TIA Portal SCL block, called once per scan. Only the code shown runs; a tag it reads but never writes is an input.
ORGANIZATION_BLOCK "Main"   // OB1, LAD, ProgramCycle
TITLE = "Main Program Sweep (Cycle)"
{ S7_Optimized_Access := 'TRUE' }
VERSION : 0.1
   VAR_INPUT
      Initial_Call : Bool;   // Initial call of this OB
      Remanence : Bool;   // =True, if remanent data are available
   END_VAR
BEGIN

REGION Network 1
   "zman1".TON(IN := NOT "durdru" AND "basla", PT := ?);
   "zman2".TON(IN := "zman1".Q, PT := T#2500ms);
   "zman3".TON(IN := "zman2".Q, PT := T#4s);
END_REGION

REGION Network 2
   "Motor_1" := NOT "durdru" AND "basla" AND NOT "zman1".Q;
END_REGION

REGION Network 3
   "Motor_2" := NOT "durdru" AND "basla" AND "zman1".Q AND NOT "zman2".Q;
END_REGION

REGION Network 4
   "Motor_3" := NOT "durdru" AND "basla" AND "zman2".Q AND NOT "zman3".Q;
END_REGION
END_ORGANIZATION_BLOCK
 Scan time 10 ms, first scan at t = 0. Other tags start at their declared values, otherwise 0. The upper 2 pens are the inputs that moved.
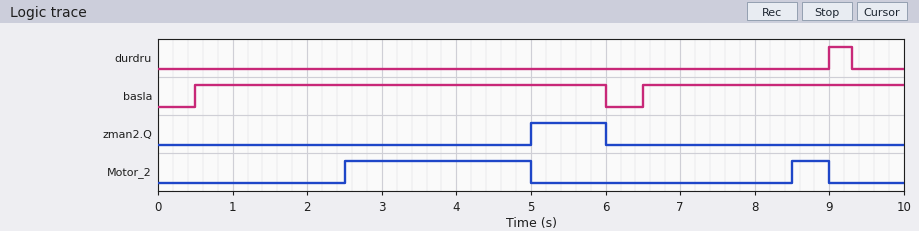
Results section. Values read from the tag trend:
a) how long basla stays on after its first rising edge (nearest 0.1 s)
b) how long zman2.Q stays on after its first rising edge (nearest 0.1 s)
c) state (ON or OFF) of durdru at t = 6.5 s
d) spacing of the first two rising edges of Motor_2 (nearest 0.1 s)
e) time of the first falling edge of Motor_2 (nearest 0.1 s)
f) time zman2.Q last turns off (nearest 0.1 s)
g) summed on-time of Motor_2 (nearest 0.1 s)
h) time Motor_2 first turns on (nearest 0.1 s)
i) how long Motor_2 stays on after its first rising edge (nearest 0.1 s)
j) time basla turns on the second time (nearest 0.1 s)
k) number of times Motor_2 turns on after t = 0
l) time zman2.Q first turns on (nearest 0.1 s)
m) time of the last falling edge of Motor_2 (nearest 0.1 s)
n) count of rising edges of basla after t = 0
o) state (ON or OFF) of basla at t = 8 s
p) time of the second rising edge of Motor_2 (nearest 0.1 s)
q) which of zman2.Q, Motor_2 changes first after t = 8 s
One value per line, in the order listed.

5.5 s
1.0 s
OFF
6.0 s
5.0 s
6.0 s
3.0 s
2.5 s
2.5 s
6.5 s
2
5.0 s
9.0 s
2
ON
8.5 s
Motor_2
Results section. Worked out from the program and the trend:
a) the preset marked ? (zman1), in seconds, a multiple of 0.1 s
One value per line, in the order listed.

2.0 s
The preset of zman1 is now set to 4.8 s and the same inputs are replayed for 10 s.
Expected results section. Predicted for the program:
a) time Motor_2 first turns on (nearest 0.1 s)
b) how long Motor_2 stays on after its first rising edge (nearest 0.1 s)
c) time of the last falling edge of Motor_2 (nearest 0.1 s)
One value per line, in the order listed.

5.3 s
0.7 s
6.0 s
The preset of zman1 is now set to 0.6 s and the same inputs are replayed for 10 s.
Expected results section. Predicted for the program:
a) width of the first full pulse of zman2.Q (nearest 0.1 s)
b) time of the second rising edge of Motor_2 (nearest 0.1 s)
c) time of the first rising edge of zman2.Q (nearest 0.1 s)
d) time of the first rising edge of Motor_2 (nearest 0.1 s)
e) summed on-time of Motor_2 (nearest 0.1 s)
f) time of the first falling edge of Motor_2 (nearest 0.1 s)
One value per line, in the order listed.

2.4 s
7.1 s
3.6 s
1.1 s
4.5 s
3.6 s
